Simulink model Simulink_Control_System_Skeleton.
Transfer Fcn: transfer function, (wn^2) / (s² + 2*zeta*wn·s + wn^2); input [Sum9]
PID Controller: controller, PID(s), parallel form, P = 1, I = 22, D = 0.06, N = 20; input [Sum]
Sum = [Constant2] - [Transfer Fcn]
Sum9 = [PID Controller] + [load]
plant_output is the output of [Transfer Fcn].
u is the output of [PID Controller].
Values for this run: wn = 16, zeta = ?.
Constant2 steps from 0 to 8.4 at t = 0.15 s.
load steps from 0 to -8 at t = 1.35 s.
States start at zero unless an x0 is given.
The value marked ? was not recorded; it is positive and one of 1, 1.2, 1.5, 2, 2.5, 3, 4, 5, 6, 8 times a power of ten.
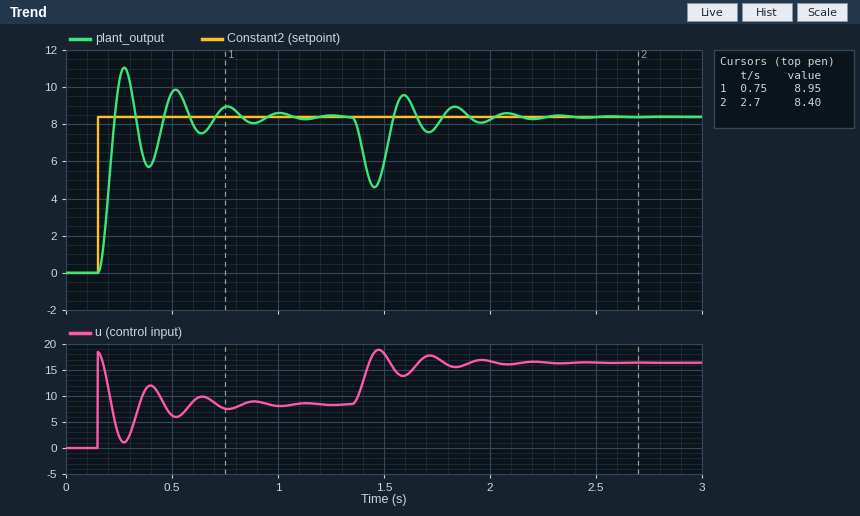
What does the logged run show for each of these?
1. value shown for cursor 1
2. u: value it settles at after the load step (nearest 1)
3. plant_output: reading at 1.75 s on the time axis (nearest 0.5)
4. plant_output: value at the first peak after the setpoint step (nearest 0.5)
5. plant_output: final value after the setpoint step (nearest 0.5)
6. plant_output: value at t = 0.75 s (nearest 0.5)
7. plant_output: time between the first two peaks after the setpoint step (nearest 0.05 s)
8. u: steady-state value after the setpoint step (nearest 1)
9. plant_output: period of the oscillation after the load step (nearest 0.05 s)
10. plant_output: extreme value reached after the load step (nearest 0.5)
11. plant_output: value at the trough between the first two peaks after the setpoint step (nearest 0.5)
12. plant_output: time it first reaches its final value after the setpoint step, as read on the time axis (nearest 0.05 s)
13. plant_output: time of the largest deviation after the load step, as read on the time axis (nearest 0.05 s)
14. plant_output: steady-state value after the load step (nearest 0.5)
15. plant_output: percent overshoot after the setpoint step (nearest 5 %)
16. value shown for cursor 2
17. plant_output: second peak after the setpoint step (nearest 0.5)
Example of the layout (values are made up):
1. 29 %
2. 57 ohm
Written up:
1. 8.95
2. 16
3. 8.0
4. 11.0
5. 8.5
6. 9.0
7. 0.25 s
8. 8
9. 0.25 s
10. 4.5
11. 5.5
12. 0.25 s
13. 1.45 s
14. 8.5
15. 30 %
16. 8.40
17. 10.0
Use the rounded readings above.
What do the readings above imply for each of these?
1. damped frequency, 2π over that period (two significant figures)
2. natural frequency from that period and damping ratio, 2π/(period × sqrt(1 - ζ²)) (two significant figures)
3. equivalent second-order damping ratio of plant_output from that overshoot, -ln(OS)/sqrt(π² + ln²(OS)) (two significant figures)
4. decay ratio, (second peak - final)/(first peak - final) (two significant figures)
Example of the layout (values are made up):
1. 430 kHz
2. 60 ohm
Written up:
1. 25 rad/s
2. 27 rad/s
3. 0.36
4. 0.60
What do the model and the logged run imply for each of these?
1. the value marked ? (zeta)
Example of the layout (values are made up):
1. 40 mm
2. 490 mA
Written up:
1. 0.3
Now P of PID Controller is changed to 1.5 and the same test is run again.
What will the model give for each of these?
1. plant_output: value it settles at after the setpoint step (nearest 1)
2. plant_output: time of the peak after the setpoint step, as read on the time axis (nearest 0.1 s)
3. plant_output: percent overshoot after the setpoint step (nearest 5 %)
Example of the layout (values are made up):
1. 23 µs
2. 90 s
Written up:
1. 8
2. 0.3 s
3. 35 %
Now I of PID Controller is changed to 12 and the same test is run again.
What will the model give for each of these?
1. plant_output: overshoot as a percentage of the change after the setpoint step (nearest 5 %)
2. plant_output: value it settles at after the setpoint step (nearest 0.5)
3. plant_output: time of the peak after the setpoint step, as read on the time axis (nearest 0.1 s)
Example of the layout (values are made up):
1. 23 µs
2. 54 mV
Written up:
1. 10 %
2. 8.5
3. 0.3 s
